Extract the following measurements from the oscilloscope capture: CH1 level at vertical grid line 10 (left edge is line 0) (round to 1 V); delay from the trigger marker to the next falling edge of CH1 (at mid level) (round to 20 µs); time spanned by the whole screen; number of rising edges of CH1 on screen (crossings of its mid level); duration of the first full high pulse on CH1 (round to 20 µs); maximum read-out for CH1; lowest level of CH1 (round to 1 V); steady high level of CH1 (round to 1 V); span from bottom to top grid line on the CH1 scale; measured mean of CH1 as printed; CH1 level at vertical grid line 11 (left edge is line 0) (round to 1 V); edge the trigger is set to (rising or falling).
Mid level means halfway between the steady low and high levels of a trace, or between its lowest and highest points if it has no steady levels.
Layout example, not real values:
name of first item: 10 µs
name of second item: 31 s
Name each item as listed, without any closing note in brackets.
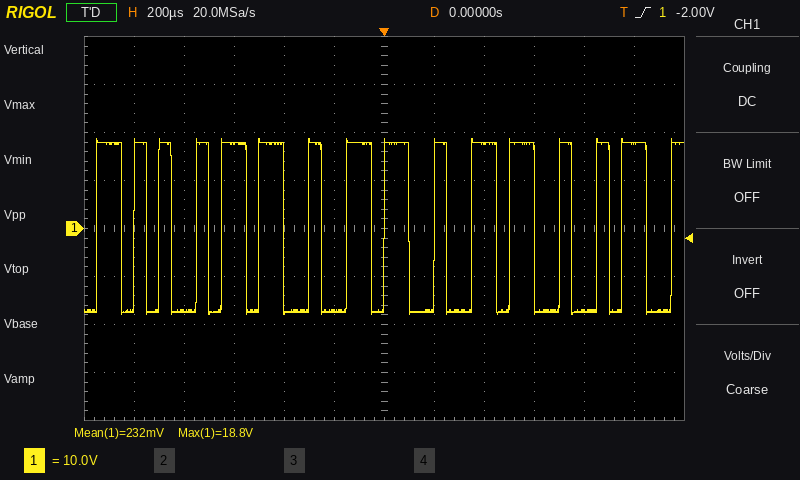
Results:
CH1 level at vertical grid line 10 (left edge is line 0): -17 V
delay from the trigger marker to the next falling edge of CH1 (at mid level): 100 µs
time spanned by the whole screen: 2.4 ms
number of rising edges of CH1 on screen: 16
duration of the first full high pulse on CH1: 100 µs
maximum read-out for CH1: 18.8 V
lowest level of CH1: -18 V
steady high level of CH1: 18 V
span from bottom to top grid line on the CH1 scale: 80 V
measured mean of CH1 as printed: 232 mV
CH1 level at vertical grid line 11 (left edge is line 0): 18 V
edge the trigger is set to: rising
